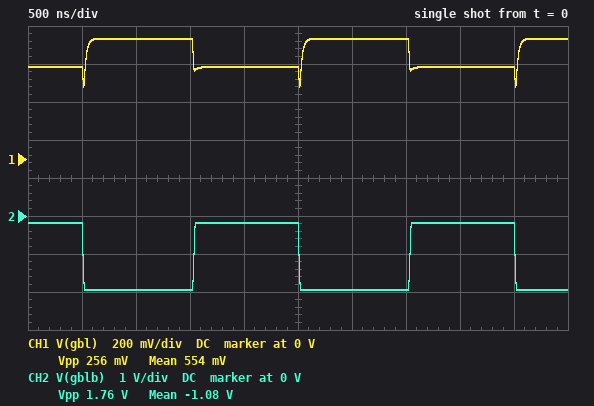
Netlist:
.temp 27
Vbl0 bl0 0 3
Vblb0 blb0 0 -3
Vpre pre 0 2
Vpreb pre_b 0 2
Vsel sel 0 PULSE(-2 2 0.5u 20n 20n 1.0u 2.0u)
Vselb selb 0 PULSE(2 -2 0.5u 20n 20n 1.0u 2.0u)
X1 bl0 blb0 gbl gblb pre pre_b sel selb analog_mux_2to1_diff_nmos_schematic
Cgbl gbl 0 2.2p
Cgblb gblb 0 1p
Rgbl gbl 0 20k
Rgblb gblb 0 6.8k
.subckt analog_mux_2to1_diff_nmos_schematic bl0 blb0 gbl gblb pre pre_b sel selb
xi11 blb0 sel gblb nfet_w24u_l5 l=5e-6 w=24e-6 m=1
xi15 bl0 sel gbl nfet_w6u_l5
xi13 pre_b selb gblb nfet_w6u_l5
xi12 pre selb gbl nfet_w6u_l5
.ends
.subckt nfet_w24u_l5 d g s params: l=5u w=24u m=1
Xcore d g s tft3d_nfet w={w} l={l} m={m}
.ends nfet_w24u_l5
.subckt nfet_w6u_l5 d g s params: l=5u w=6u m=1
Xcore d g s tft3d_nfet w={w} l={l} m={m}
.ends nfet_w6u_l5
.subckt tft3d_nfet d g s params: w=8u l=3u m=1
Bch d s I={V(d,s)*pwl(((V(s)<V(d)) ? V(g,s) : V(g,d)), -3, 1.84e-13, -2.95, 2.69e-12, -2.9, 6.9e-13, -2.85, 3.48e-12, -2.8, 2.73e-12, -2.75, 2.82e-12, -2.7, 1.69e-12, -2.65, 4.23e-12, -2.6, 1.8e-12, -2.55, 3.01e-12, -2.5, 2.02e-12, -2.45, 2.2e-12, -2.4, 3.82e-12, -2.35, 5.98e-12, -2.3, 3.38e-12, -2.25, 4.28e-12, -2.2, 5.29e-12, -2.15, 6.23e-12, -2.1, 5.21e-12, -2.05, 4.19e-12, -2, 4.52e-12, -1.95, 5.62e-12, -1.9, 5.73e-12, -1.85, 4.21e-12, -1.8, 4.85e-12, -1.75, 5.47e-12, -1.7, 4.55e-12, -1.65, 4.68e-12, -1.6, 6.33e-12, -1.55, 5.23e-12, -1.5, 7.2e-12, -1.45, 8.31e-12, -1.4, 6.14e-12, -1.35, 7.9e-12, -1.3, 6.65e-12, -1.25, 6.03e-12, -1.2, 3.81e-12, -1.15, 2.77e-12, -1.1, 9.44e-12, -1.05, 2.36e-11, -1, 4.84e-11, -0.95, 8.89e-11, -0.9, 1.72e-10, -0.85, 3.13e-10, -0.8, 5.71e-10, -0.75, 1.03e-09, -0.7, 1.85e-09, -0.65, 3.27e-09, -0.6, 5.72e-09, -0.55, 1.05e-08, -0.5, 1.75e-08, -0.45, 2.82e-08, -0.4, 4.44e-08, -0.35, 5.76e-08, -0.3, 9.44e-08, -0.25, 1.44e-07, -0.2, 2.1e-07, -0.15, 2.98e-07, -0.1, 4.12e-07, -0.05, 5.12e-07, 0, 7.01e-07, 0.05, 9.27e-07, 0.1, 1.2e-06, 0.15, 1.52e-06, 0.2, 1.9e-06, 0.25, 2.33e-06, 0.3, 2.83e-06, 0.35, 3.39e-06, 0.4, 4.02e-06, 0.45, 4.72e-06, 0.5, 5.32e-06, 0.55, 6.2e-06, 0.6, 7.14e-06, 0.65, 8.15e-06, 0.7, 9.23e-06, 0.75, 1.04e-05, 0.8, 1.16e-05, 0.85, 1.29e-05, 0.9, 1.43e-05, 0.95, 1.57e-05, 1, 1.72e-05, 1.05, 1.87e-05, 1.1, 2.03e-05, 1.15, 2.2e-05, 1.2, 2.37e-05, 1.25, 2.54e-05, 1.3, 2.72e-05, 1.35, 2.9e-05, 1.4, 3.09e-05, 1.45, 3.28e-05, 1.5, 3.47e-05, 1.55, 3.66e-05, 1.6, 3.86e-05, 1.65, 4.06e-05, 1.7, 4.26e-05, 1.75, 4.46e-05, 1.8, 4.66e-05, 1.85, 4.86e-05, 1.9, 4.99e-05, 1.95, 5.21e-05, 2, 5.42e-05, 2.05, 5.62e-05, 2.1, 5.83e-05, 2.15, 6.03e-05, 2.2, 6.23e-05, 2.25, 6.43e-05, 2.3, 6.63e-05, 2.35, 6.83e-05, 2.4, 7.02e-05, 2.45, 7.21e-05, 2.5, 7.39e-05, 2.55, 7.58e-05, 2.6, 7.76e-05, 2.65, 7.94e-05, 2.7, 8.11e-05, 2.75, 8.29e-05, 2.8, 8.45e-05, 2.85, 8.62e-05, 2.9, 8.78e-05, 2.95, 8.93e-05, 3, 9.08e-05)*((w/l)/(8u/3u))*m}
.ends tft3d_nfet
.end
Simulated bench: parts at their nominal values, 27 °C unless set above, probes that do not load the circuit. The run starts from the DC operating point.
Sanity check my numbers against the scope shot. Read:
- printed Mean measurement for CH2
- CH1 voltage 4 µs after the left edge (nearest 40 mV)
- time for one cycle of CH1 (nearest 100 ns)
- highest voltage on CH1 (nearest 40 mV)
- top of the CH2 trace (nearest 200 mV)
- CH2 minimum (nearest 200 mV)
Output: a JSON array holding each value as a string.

["-1.08 V", "480 mV", "2.0 µs", "640 mV", "-200 mV", "-2.0 V"]
